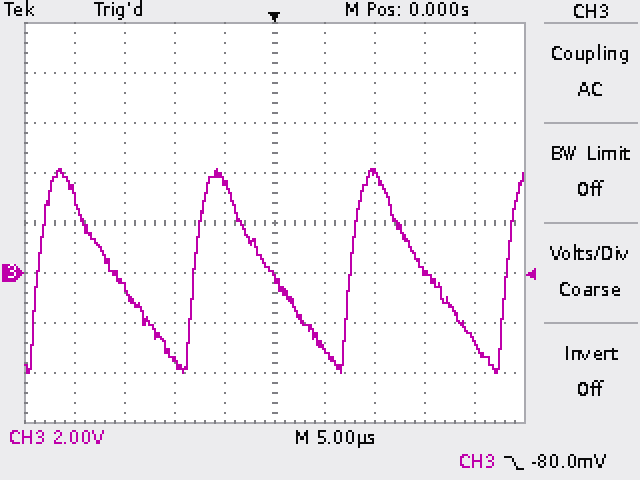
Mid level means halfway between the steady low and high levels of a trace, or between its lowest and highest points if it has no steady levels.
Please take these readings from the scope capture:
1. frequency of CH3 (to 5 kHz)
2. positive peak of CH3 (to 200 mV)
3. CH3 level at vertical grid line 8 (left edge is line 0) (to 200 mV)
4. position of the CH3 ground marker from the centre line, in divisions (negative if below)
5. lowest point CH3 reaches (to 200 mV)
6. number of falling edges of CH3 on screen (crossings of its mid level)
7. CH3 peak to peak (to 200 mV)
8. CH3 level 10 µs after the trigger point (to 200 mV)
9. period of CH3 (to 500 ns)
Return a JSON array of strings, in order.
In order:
["65 kHz", "4.2 V", "0.0 V", "-1.0 div", "-4.0 V", "3", "8.2 V", "4.0 V", "15.5 µs"]
